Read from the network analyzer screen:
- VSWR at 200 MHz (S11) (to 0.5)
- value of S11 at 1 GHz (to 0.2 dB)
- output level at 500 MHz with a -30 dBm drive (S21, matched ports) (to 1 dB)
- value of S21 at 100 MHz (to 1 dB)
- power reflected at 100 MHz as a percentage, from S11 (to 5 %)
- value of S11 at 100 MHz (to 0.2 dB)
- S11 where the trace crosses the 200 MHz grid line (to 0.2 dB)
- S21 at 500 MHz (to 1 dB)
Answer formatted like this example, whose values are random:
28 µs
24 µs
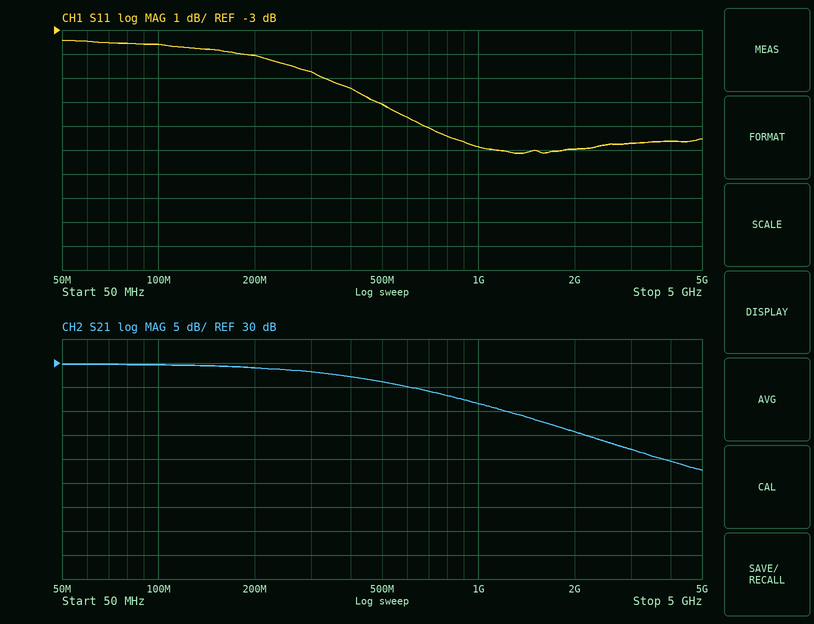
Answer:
4.5
-7.8 dB
-4 dBm
30 dB
45 %
-3.6 dB
-4.0 dB
26 dB
